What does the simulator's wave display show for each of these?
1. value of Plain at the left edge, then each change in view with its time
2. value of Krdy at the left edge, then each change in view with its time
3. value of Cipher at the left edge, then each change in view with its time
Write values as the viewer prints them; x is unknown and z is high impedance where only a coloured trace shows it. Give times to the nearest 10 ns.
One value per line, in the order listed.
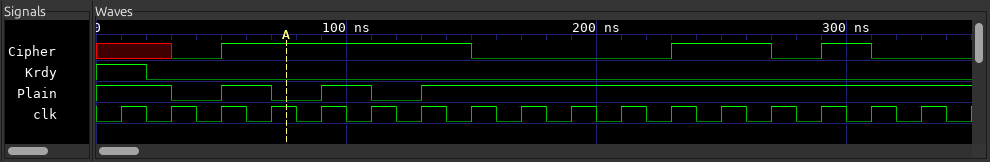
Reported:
1, 0 at 30 ns, 1 at 50 ns, 0 at 70 ns, 1 at 90 ns, 0 at 110 ns, 1 at 130 ns
1, 0 at 20 ns
x, 0 at 30 ns, 1 at 50 ns, 0 at 150 ns, 1 at 230 ns, 0 at 270 ns, 1 at 290 ns, 0 at 310 ns
